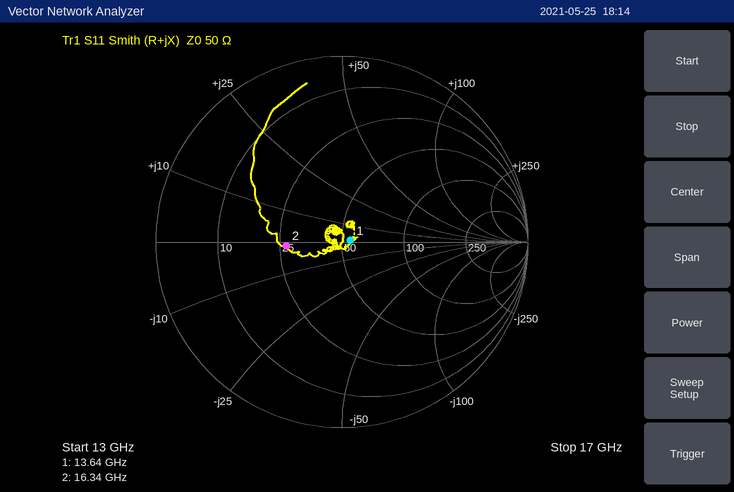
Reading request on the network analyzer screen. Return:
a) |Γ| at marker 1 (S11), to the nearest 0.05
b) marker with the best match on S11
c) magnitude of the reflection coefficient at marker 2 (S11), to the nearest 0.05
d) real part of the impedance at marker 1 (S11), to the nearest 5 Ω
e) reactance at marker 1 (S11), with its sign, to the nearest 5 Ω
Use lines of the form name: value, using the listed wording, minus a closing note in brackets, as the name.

|Γ| at marker 1 (S11), to the nearest 0.05: 0.05
marker with the best match on S11: marker 1
magnitude of the reflection coefficient at marker 2 (S11), to the nearest 0.05: 0.30
real part of the impedance at marker 1 (S11), to the nearest 5 Ω: 55 Ω
reactance at marker 1 (S11), with its sign, to the nearest 5 Ω: 0 Ω
